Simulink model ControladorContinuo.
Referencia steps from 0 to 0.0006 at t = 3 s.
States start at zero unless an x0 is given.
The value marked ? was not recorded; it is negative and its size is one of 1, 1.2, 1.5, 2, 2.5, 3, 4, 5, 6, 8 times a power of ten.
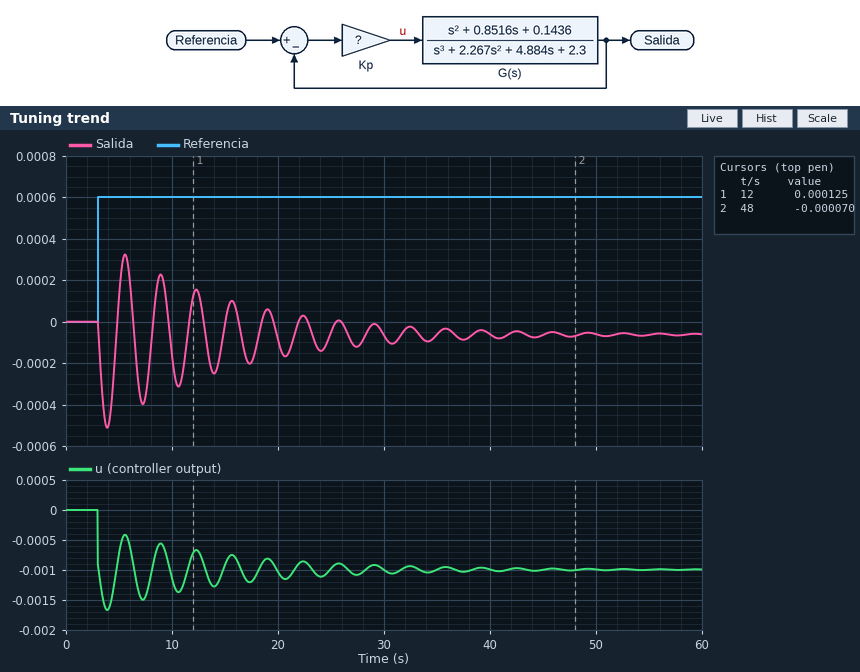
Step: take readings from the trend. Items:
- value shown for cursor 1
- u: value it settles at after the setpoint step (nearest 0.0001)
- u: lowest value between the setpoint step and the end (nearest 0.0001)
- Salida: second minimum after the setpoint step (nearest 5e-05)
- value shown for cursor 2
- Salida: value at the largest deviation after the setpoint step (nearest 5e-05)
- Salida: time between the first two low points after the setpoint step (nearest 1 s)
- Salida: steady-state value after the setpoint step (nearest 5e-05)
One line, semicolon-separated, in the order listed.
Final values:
0.000125; -0.0010; -0.0017; -0.00040; -0.000070; -0.00050; 3 s; -0.00005
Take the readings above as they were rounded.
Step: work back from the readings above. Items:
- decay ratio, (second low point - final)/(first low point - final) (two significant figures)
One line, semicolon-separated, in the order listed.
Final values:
0.78
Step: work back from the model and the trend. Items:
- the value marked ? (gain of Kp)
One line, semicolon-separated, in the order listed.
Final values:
-1.5
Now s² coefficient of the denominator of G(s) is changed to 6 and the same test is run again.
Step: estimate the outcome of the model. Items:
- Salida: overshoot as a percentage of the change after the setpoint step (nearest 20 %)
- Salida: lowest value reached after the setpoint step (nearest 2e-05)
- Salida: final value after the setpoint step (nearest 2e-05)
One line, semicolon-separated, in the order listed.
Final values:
260 %; -0.00022; -0.00006
